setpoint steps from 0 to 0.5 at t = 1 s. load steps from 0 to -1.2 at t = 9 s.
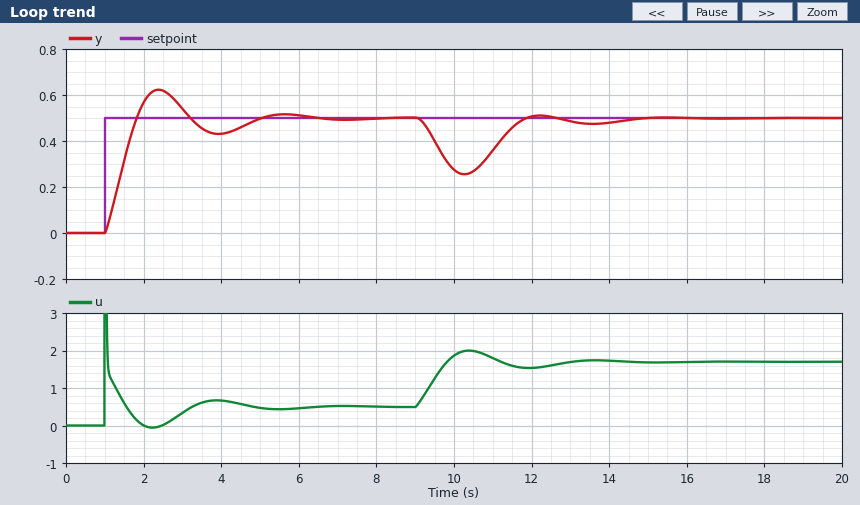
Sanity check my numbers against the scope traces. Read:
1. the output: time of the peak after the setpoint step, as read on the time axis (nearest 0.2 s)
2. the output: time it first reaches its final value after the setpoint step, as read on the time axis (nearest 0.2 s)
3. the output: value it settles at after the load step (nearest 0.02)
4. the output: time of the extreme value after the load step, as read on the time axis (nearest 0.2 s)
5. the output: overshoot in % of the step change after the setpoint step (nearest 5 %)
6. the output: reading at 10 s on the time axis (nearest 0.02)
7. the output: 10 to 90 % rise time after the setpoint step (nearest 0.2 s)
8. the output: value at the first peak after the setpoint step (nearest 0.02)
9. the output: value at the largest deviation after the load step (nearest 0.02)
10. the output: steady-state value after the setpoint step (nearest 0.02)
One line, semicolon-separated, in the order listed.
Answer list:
2.4 s; 1.8 s; 0.50; 10.2 s; 25 %; 0.28; 0.6 s; 0.62; 0.26; 0.50
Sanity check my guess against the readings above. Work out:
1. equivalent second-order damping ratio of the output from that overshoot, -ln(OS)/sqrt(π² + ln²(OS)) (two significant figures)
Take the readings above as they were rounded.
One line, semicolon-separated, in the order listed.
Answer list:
0.40
